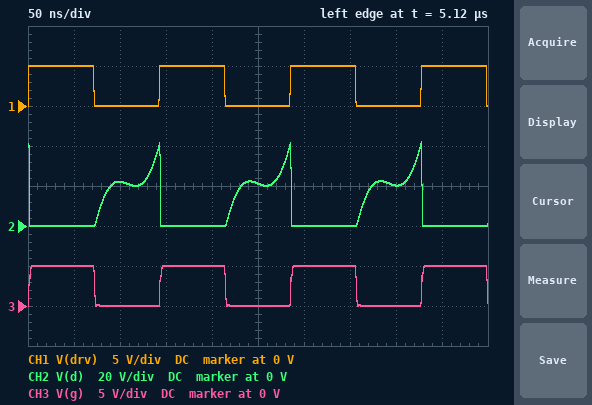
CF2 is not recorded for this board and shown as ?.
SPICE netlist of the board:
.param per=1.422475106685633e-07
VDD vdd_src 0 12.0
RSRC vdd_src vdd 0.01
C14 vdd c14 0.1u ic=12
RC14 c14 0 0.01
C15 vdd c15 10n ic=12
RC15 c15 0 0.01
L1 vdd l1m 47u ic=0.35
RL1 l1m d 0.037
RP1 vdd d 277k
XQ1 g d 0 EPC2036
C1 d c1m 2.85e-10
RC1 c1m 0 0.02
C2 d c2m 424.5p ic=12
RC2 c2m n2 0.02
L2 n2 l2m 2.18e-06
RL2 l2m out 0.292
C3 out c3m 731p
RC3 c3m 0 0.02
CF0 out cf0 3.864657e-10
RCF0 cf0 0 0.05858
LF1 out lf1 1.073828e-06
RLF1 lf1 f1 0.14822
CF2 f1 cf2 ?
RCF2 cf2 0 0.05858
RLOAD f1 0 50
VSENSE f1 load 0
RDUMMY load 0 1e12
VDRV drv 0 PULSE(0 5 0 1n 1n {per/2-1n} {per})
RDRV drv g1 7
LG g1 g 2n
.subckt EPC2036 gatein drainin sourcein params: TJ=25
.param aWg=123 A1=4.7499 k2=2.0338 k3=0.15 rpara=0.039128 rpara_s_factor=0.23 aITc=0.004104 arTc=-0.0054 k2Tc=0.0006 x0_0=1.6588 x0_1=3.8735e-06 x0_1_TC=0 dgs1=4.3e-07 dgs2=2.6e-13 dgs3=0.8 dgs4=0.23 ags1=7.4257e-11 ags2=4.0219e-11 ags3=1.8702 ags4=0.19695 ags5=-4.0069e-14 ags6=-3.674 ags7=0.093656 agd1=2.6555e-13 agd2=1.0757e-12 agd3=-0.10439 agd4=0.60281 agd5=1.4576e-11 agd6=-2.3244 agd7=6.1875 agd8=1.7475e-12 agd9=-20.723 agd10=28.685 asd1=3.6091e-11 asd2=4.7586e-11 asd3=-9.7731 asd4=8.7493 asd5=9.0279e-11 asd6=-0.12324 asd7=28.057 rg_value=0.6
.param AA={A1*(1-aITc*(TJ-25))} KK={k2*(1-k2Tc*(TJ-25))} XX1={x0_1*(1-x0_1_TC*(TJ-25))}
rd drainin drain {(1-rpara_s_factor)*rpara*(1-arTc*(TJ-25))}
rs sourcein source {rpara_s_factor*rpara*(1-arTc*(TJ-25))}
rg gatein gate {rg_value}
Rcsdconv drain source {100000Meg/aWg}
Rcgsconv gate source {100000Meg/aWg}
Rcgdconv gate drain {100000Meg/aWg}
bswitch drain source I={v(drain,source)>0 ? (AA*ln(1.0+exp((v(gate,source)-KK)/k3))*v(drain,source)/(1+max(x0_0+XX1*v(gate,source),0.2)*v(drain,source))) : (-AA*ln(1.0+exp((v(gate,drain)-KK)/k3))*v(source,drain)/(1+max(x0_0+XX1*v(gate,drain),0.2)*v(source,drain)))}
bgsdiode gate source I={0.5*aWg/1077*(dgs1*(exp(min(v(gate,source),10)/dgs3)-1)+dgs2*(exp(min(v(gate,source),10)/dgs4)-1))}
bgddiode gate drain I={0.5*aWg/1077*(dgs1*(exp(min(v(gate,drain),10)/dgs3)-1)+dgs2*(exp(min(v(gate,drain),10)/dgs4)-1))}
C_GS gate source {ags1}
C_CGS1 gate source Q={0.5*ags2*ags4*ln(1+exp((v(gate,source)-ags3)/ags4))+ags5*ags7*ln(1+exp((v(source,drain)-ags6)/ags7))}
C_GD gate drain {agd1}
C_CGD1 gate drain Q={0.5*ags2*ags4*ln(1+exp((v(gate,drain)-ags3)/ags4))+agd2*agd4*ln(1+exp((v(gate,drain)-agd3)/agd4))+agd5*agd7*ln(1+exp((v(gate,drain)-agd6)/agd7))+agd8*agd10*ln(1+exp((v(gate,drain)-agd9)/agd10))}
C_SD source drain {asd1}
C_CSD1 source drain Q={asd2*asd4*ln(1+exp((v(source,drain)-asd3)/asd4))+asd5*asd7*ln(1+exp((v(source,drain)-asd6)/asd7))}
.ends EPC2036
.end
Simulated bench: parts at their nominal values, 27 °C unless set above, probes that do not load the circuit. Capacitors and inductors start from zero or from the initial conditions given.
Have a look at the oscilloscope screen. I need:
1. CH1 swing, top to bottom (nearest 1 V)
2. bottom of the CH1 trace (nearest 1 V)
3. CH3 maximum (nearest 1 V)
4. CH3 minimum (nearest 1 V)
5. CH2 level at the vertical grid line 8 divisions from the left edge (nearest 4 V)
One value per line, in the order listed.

5 V
0 V
5 V
0 V
20 V
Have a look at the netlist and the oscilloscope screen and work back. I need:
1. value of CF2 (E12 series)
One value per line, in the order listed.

1.2 nF
